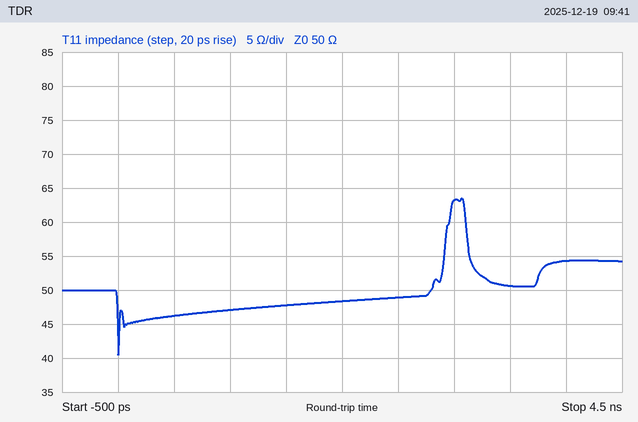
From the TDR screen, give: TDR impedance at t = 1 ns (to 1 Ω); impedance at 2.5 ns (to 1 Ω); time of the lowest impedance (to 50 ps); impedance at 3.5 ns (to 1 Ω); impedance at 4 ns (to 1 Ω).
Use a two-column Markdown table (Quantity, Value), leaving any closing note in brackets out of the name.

| Quantity | Value |
|---|---|
| TDR impedance at t = 1 ns | 47 Ω |
| impedance at 2.5 ns | 49 Ω |
| time of the lowest impedance | 0 ps |
| impedance at 3.5 ns | 51 Ω |
| impedance at 4 ns | 54 Ω |
